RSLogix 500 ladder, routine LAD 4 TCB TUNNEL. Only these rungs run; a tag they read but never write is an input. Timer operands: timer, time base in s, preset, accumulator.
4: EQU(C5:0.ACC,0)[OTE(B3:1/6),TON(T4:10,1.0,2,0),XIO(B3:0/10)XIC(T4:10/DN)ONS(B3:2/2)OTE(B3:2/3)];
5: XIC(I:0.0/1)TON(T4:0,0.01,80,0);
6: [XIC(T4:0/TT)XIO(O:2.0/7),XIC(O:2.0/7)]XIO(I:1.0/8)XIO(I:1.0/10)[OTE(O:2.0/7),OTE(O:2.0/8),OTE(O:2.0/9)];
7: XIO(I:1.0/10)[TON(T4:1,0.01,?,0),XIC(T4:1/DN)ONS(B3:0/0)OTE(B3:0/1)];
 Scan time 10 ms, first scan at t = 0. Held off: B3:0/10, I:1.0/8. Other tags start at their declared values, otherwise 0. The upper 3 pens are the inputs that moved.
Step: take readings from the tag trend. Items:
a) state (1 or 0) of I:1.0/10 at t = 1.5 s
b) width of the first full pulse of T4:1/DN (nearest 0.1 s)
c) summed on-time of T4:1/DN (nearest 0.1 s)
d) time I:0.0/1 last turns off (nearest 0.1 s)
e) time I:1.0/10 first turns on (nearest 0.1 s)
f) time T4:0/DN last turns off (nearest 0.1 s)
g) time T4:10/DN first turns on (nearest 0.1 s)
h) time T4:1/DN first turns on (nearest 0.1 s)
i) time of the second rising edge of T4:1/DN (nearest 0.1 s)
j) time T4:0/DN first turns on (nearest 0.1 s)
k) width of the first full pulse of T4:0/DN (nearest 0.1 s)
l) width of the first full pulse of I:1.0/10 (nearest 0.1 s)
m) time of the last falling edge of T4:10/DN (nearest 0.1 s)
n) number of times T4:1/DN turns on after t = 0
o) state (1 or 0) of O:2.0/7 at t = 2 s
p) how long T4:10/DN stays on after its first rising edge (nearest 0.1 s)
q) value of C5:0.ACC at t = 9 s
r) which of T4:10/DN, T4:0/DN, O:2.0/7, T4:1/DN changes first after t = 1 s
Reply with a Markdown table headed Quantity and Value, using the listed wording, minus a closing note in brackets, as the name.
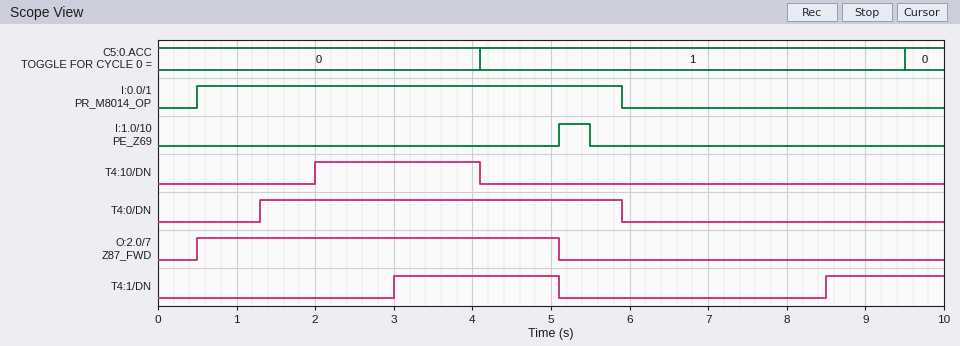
| Quantity | Value |
|---|---|
| state (1 or 0) of I:1.0/10 at t = 1.5 s | 0 |
| width of the first full pulse of T4:1/DN | 2.1 s |
| summed on-time of T4:1/DN | 3.6 s |
| time I:0.0/1 last turns off | 5.9 s |
| time I:1.0/10 first turns on | 5.1 s |
| time T4:0/DN last turns off | 5.9 s |
| time T4:10/DN first turns on | 2.0 s |
| time T4:1/DN first turns on | 3.0 s |
| time of the second rising edge of T4:1/DN | 8.5 s |
| time T4:0/DN first turns on | 1.3 s |
| width of the first full pulse of T4:0/DN | 4.6 s |
| width of the first full pulse of I:1.0/10 | 0.4 s |
| time of the last falling edge of T4:10/DN | 4.1 s |
| number of times T4:1/DN turns on after t = 0 | 2 |
| state (1 or 0) of O:2.0/7 at t = 2 s | 1 |
| how long T4:10/DN stays on after its first rising edge | 2.1 s |
| value of C5:0.ACC at t = 9 s | 1 |
| which of T4:10/DN, T4:0/DN, O:2.0/7, T4:1/DN changes first after t = 1 s | T4:0/DN |
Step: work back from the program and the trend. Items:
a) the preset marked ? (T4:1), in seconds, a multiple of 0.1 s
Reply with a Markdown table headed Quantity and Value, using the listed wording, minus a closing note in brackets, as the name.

| Quantity | Value |
|---|---|
| the preset marked ? (T4:1), in seconds, a multiple of 0.1 s | 3.0 s |
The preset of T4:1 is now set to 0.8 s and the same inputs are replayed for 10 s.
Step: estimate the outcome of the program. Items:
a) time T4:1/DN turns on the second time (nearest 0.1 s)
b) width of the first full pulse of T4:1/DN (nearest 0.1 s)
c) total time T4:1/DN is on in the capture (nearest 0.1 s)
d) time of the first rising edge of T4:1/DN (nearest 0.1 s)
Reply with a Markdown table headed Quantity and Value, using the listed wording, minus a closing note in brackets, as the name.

| Quantity | Value |
|---|---|
| time T4:1/DN turns on the second time | 6.3 s |
| width of the first full pulse of T4:1/DN | 4.3 s |
| total time T4:1/DN is on in the capture | 8.0 s |
| time of the first rising edge of T4:1/DN | 0.8 s |
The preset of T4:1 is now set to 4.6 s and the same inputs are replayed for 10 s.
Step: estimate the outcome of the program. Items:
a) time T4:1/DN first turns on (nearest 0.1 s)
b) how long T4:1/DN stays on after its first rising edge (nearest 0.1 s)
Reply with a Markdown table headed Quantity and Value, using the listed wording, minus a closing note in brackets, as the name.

| Quantity | Value |
|---|---|
| time T4:1/DN first turns on | 4.6 s |
| how long T4:1/DN stays on after its first rising edge | 0.5 s |
